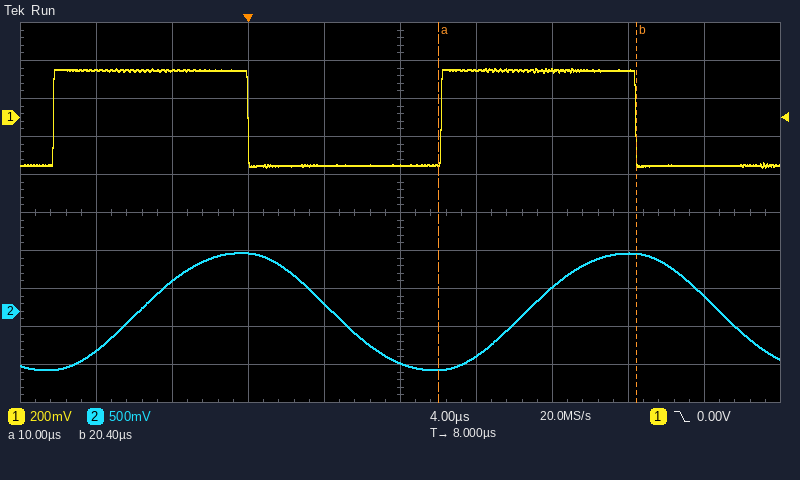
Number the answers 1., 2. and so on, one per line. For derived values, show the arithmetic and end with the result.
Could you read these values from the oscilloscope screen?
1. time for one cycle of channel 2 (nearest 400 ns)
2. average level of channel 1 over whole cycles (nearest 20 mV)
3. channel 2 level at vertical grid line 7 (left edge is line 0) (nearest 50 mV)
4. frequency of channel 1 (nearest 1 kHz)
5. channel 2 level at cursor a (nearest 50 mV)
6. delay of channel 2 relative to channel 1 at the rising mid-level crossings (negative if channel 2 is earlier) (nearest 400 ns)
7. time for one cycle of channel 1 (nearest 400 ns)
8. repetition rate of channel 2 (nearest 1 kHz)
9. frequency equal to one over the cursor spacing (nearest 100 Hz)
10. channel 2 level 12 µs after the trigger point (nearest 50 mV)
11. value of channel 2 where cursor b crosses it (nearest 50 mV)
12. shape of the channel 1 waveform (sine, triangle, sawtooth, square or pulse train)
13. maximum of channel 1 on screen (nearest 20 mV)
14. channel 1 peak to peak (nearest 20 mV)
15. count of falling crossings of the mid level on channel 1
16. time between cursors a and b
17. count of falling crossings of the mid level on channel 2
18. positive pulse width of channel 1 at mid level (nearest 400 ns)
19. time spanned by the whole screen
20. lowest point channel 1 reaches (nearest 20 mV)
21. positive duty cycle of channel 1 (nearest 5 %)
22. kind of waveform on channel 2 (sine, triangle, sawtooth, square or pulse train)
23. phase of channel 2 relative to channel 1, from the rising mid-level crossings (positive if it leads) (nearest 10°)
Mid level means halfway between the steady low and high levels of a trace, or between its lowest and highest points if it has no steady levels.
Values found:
1. 20.4 µs
2. -260 mV + 0.5 × (260 mV − (-260 mV)) ≈ 0 mV
3. 300 mV
4. 1 / 20.4 µs ≈ 49 kHz
5. -750 mV
6. +4.4 µs
7. 20.4 µs
8. 1 / 20.4 µs ≈ 49 kHz
9. 1 / 10.4 µs ≈ 96.2 kHz
10. -600 mV
11. 750 mV
12. square
13. 260 mV
14. 260 mV − (-260 mV) = 520 mV
15. 2
16. 20.4 µs − (10 µs) = 10.4 µs
17. 2
18. 10.4 µs
19. 40 µs
20. -260 mV
21. 10.4 µs / 20.4 µs ≈ 51.0 %, so 50 % to the nearest 5 %
22. sine
23. −360° × (+4.4 µs) / 20.4 µs ≈ -77.6°, so -80° to the nearest 10°
